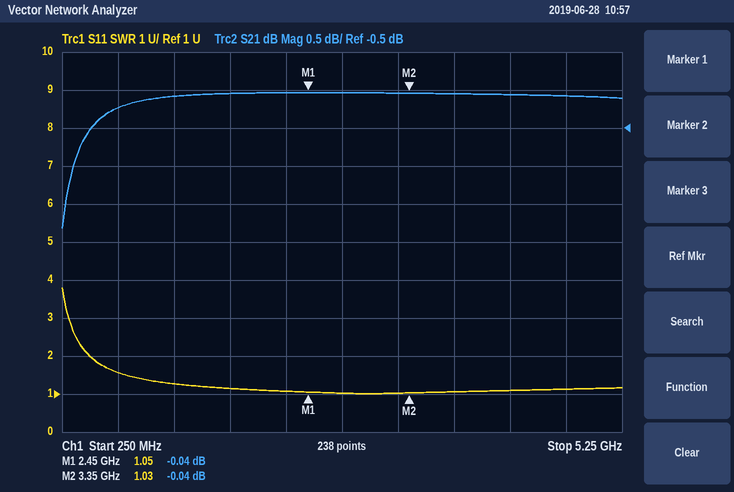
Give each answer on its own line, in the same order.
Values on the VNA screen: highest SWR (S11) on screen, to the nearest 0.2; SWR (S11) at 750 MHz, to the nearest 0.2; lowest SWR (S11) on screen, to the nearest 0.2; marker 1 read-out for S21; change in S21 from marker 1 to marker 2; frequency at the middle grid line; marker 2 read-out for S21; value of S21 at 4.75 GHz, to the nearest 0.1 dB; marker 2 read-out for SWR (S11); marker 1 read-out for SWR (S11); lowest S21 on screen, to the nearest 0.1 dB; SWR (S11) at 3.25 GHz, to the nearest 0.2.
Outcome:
3.8
1.6
1.0
-0.04 dB
0.00 dB
2.75 GHz
-0.04 dB
-0.1 dB
1.03
1.05
-1.8 dB
1.0
